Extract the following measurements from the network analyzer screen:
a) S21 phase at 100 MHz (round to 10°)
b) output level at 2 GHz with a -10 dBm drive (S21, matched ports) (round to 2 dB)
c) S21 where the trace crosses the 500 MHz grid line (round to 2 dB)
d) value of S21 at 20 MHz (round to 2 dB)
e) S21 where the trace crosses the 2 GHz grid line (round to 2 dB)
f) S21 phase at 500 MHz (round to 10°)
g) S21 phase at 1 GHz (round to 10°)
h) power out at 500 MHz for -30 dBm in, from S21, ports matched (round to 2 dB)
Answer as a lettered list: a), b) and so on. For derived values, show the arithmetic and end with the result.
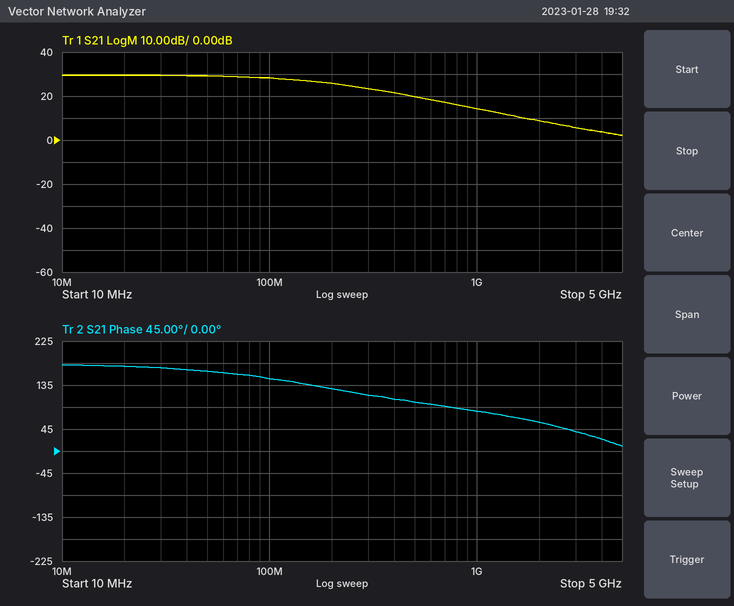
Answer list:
a) 150°
b) -10 dBm + (8 dB) = -2 dBm
c) 20 dB
d) 30 dB
e) 8 dB
f) 100°
g) 80°
h) -30 dBm + (20 dB) = -10 dBm
